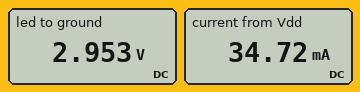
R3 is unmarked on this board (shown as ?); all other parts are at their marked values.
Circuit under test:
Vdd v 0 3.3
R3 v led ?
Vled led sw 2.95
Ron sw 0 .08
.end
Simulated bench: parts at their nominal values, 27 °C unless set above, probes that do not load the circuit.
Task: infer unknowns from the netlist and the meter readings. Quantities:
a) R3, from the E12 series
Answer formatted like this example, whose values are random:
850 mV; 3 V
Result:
10 Ω
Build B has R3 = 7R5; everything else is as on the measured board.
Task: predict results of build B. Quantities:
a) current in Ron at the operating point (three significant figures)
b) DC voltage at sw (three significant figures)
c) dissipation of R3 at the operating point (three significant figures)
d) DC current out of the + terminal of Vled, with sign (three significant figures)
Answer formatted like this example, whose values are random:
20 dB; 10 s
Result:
46.2 mA; 3.69 mV; 16.0 mW; -46.2 mA
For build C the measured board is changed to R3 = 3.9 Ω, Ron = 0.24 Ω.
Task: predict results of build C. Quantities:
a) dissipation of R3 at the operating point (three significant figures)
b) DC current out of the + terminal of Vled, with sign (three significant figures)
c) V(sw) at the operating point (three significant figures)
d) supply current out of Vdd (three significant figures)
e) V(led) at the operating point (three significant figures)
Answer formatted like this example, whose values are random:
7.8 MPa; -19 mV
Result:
27.9 mW; -84.5 mA; 20.3 mV; 84.5 mA; 2.97 V
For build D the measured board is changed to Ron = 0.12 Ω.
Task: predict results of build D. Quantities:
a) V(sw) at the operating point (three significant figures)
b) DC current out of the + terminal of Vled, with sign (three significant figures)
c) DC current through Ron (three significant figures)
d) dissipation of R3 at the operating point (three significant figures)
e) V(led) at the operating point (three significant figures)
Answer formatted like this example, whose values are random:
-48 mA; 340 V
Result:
4.15 mV; -34.6 mA; 34.6 mA; 12.0 mW; 2.95 V
